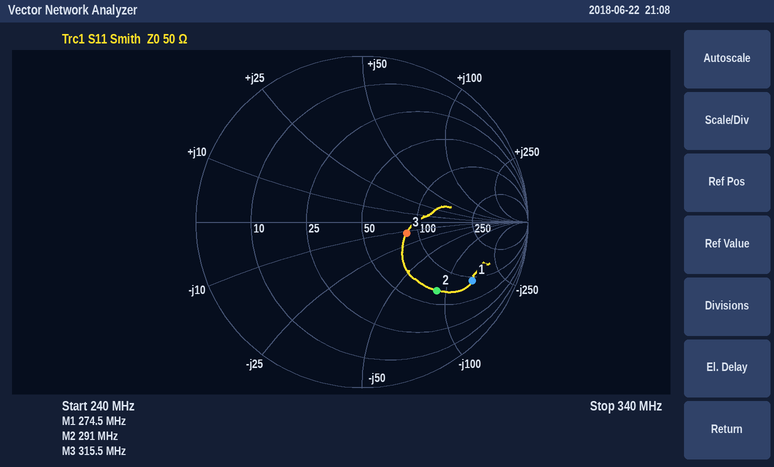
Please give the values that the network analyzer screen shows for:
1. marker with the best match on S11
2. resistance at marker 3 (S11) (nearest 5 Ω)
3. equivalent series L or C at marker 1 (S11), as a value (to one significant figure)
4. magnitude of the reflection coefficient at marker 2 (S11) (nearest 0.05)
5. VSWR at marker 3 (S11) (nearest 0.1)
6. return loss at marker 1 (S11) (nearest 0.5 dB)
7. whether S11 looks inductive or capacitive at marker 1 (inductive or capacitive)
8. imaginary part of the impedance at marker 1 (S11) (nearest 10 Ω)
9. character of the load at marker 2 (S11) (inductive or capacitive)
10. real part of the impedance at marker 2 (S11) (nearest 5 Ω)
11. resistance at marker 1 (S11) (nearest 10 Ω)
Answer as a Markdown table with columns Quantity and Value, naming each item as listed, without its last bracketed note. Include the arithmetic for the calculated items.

| Quantity | Value |
|---|---|
| marker with the best match on S11 | marker 3 |
| resistance at marker 3 (S11) | 85 Ω |
| equivalent series L or C at marker 1 (S11), as a value | C = 1/(2π × 274.5 MHz × 150 Ω) ≈ 4 pF |
| magnitude of the reflection coefficient at marker 2 (S11) | 0.60 |
| VSWR at marker 3 (S11) | 1.8 |
| return loss at marker 1 (S11) | 2.5 dB |
| whether S11 looks inductive or capacitive at marker 1 | capacitive |
| imaginary part of the impedance at marker 1 (S11) | -150 Ω |
| character of the load at marker 2 (S11) | capacitive |
| real part of the impedance at marker 2 (S11) | 65 Ω |
| resistance at marker 1 (S11) | 90 Ω |
